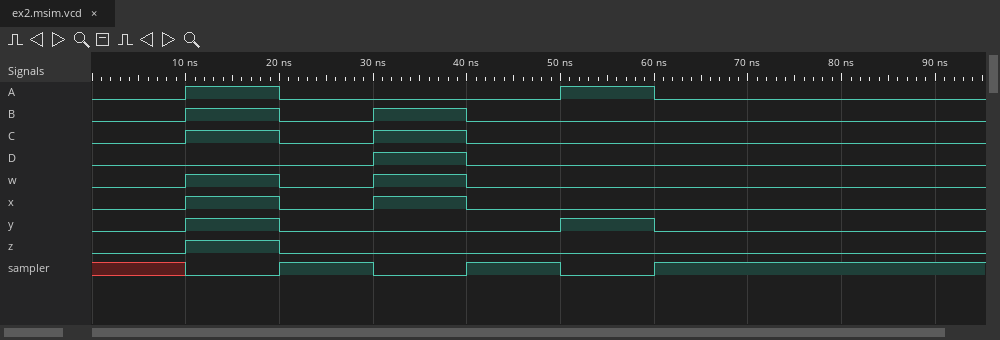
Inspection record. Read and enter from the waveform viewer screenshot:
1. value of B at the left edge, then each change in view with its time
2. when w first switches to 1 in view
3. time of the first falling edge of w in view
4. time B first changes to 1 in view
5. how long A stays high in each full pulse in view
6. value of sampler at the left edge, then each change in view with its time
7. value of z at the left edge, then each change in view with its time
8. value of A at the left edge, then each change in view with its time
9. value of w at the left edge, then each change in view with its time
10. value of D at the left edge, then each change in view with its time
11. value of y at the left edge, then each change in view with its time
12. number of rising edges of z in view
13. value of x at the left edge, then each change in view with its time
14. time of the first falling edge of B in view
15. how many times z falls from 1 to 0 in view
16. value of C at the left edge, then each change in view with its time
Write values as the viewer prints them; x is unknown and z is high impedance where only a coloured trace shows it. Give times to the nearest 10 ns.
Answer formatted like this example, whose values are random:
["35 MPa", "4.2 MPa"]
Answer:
["0, 1 at 10 ns, 0 at 20 ns, 1 at 30 ns, 0 at 40 ns", "10 ns", "20 ns", "10 ns", "10 ns, 10 ns", "x, 0 at 10 ns, 1 at 20 ns, 0 at 30 ns, 1 at 40 ns, 0 at 50 ns, 1 at 60 ns", "0, 1 at 10 ns, 0 at 20 ns", "0, 1 at 10 ns, 0 at 20 ns, 1 at 50 ns, 0 at 60 ns", "0, 1 at 10 ns, 0 at 20 ns, 1 at 30 ns, 0 at 40 ns", "0, 1 at 30 ns, 0 at 40 ns", "0, 1 at 10 ns, 0 at 20 ns, 1 at 50 ns, 0 at 60 ns", "1", "0, 1 at 10 ns, 0 at 20 ns, 1 at 30 ns, 0 at 40 ns", "20 ns", "1", "0, 1 at 10 ns, 0 at 20 ns, 1 at 30 ns, 0 at 40 ns"]
